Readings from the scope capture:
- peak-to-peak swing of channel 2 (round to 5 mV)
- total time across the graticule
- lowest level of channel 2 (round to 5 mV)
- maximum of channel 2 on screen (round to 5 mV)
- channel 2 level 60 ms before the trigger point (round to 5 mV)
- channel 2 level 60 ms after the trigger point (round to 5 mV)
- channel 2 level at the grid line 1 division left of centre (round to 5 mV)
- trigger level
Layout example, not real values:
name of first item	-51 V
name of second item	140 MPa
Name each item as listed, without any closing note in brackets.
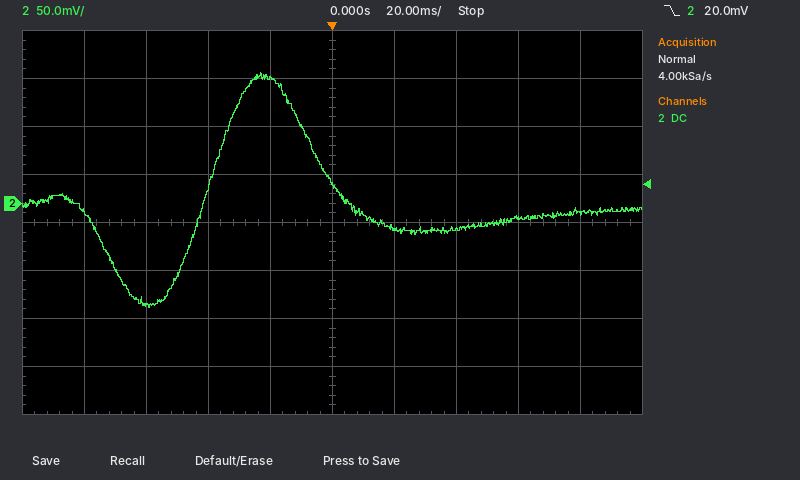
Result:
peak-to-peak swing of channel 2	245 mV
total time across the graticule	200 ms
lowest level of channel 2	-110 mV
maximum of channel 2 on screen	135 mV
channel 2 level 60 ms before the trigger point	-105 mV
channel 2 level 60 ms after the trigger point	-15 mV
channel 2 level at the grid line 1 division left of centre	130 mV
trigger level	20.0 mV
